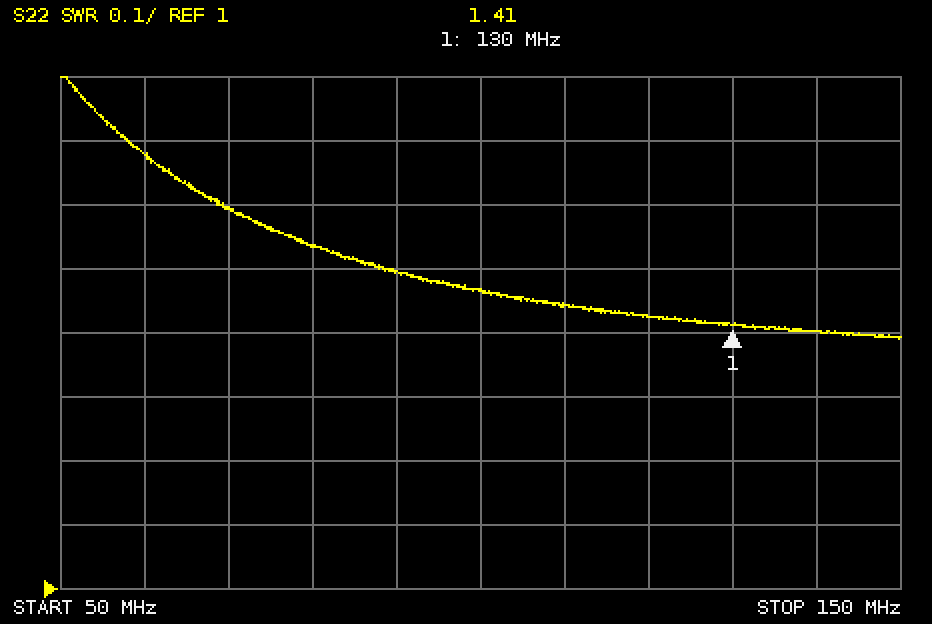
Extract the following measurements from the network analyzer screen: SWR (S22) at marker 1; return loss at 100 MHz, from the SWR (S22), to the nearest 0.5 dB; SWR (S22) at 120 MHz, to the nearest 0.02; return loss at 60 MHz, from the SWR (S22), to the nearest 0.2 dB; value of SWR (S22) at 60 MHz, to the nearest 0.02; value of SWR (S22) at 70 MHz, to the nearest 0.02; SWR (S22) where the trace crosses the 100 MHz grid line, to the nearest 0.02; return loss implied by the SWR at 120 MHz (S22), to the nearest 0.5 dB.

1.41
14.5 dB
1.42
12.0 dB
1.68
1.60
1.46
15.0 dB
